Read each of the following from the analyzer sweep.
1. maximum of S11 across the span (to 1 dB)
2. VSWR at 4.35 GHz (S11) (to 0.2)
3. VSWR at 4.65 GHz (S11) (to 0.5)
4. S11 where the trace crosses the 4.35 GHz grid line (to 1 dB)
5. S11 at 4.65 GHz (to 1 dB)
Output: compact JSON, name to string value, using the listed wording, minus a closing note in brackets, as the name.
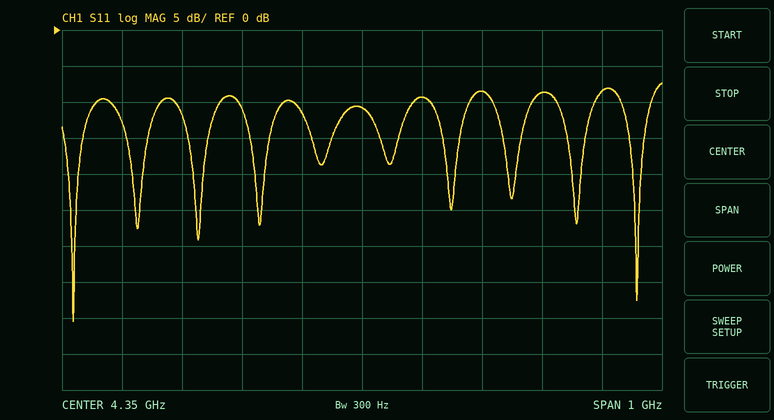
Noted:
{"maximum of S11 across the span": "-7 dB", "VSWR at 4.35 GHz (S11)": "1.8", "VSWR at 4.65 GHz (S11)": "2.0", "S11 where the trace crosses the 4.35 GHz grid line": "-11 dB", "S11 at 4.65 GHz": "-9 dB"}
